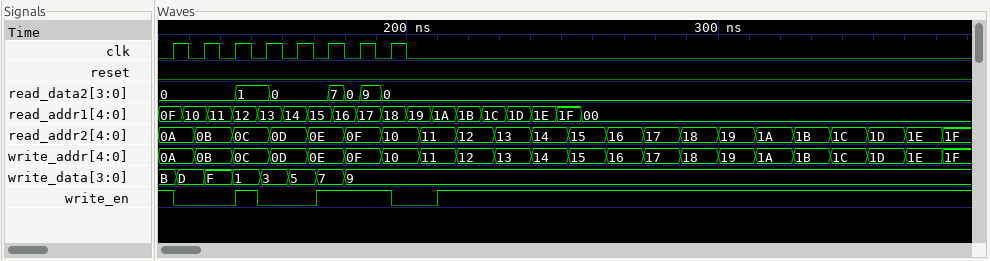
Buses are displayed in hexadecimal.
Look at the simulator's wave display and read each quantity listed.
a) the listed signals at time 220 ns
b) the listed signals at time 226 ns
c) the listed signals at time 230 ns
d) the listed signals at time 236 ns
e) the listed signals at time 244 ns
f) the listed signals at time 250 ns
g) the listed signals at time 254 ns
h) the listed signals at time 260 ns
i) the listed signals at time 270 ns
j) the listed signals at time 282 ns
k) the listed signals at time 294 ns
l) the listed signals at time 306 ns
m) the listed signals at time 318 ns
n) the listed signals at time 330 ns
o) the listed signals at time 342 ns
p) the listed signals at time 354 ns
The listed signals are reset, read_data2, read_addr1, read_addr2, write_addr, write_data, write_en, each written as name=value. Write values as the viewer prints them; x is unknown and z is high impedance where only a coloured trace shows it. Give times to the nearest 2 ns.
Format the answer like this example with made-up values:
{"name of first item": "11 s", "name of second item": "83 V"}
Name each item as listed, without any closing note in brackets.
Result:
{"the listed signals at time 220 ns": "reset=0, read_data2=0, read_addr1=1B, read_addr2=12, write_addr=12, write_data=9, write_en=1", "the listed signals at time 226 ns": "reset=0, read_data2=0, read_addr1=1C, read_addr2=12, write_addr=12, write_data=9, write_en=1", "the listed signals at time 230 ns": "reset=0, read_data2=0, read_addr1=1C, read_addr2=13, write_addr=13, write_data=9, write_en=1", "the listed signals at time 236 ns": "reset=0, read_data2=0, read_addr1=1D, read_addr2=13, write_addr=13, write_data=9, write_en=1", "the listed signals at time 244 ns": "reset=0, read_data2=0, read_addr1=1E, read_addr2=14, write_addr=14, write_data=9, write_en=1", "the listed signals at time 250 ns": "reset=0, read_data2=0, read_addr1=1F, read_addr2=14, write_addr=14, write_data=9, write_en=1", "the listed signals at time 254 ns": "reset=0, read_data2=0, read_addr1=1F, read_addr2=15, write_addr=15, write_data=9, write_en=1", "the listed signals at time 260 ns": "reset=0, read_data2=0, read_addr1=00, read_addr2=15, write_addr=15, write_data=9, write_en=1", "the listed signals at time 270 ns": "reset=0, read_data2=0, read_addr1=00, read_addr2=16, write_addr=16, write_data=9, write_en=1", "the listed signals at time 282 ns": "reset=0, read_data2=0, read_addr1=00, read_addr2=17, write_addr=17, write_data=9, write_en=1", "the listed signals at time 294 ns": "reset=0, read_data2=0, read_addr1=00, read_addr2=18, write_addr=18, write_data=9, write_en=1", "the listed signals at time 306 ns": "reset=0, read_data2=0, read_addr1=00, read_addr2=19, write_addr=19, write_data=9, write_en=1", "the listed signals at time 318 ns": "reset=0, read_data2=0, read_addr1=00, read_addr2=1A, write_addr=1A, write_data=9, write_en=1", "the listed signals at time 330 ns": "reset=0, read_data2=0, read_addr1=00, read_addr2=1B, write_addr=1B, write_data=9, write_en=1", "the listed signals at time 342 ns": "reset=0, read_data2=0, read_addr1=00, read_addr2=1C, write_addr=1C, write_data=9, write_en=1", "the listed signals at time 354 ns": "reset=0, read_data2=0, read_addr1=00, read_addr2=1D, write_addr=1D, write_data=9, write_en=1"}
